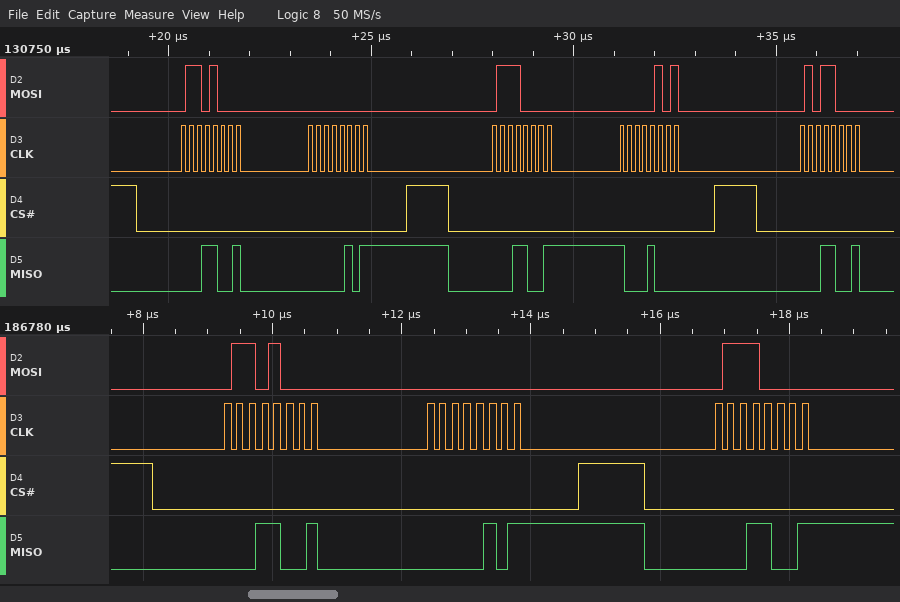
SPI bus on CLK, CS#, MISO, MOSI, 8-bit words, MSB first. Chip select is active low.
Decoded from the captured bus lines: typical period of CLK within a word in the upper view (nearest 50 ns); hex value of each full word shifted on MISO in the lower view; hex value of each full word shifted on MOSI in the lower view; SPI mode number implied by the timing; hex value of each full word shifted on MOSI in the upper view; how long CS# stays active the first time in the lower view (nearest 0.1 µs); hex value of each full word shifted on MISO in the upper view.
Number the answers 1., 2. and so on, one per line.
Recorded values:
1. 200 ns
2. 19, 05, 19
3. 68, 00, 70
4. 0
5. 68, 00, 70, 05, 58
6. 6.6 µs
7. 19, 05, 19, 88, 19
